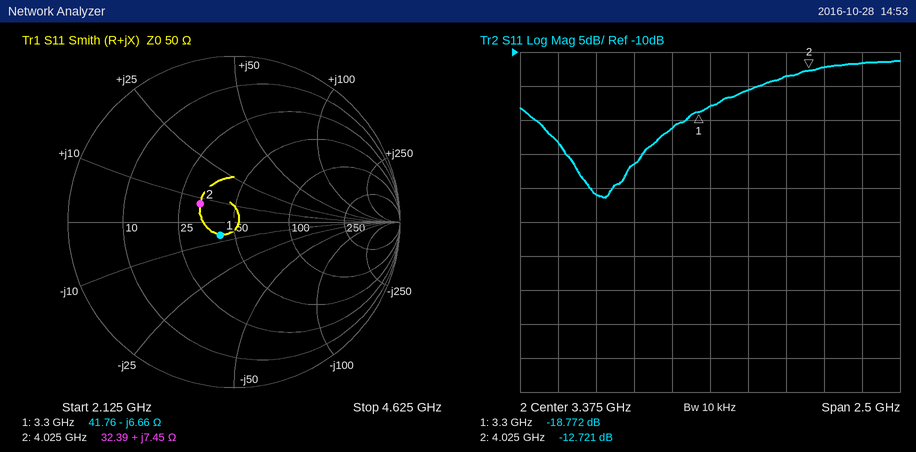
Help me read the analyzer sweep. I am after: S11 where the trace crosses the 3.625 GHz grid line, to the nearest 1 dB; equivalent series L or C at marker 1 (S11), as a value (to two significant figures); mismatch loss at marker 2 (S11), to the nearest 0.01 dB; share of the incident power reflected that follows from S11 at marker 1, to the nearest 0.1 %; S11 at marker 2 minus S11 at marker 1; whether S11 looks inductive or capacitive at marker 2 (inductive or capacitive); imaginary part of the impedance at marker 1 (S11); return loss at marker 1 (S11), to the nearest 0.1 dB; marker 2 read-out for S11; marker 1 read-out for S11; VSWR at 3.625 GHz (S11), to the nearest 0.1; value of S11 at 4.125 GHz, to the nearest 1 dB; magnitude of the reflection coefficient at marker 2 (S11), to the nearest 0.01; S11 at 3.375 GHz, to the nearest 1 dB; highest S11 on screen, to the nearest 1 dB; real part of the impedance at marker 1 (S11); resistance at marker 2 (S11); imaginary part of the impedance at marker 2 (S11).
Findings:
-16 dB
7.2 pF
0.24 dB
1.3 %
6.051 dB
inductive
-6.66 Ω
18.8 dB
-12.721 dB
-18.772 dB
1.4
-12 dB
0.23
-18 dB
-11 dB
41.76 Ω
32.39 Ω
+7.45 Ω
